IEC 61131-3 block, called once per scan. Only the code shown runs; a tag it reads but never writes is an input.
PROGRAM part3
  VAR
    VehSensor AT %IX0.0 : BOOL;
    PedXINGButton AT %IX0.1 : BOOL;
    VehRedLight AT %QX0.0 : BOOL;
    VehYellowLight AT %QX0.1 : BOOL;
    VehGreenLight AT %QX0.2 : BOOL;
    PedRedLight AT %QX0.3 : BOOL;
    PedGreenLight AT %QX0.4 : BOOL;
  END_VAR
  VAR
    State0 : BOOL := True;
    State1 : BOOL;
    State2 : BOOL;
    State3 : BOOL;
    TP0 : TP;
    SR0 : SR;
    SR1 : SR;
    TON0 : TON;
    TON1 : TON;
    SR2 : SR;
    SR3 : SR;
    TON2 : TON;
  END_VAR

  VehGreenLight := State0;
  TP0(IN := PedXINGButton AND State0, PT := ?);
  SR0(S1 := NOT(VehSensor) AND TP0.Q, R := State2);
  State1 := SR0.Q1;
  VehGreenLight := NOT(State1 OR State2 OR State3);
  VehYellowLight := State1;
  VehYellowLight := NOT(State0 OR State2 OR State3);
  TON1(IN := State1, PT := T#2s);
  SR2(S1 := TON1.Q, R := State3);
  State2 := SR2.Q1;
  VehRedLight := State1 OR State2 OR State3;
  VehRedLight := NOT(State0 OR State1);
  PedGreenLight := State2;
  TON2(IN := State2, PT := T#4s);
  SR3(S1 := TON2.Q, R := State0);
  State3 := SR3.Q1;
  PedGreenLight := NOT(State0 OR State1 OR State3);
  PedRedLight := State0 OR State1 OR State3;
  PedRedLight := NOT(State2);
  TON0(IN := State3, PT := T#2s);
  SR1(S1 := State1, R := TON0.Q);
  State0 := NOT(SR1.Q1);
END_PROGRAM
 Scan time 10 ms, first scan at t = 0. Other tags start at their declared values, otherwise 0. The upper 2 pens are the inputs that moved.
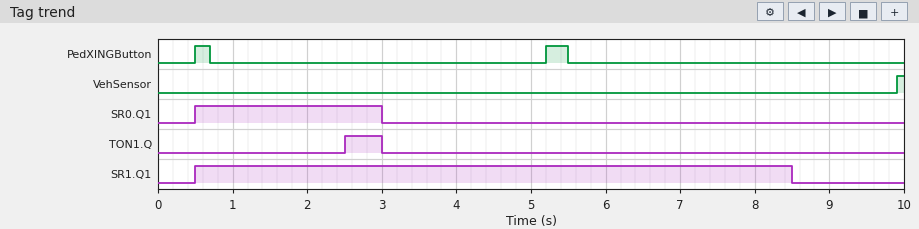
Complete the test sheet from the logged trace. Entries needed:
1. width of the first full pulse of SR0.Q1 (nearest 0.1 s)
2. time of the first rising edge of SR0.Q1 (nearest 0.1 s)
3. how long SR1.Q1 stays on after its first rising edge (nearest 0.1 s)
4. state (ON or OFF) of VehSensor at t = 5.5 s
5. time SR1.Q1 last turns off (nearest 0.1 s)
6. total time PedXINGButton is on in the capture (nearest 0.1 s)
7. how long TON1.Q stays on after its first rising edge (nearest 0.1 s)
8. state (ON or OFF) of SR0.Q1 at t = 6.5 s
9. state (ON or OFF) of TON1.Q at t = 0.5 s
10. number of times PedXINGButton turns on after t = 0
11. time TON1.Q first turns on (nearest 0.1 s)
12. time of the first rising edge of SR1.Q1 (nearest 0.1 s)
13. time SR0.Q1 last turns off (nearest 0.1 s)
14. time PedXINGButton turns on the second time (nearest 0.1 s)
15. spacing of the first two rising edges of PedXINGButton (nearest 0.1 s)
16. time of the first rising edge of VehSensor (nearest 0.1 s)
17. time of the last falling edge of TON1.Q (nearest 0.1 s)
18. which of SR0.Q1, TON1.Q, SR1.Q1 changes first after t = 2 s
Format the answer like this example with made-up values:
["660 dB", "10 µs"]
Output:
["2.5 s", "0.5 s", "8.0 s", "OFF", "8.5 s", "0.5 s", "0.5 s", "OFF", "OFF", "2", "2.5 s", "0.5 s", "3.0 s", "5.2 s", "4.7 s", "9.9 s", "3.0 s", "TON1.Q"]
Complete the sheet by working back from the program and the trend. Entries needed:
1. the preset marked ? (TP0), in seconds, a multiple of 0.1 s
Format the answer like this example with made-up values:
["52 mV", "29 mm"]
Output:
["2.5 s"]
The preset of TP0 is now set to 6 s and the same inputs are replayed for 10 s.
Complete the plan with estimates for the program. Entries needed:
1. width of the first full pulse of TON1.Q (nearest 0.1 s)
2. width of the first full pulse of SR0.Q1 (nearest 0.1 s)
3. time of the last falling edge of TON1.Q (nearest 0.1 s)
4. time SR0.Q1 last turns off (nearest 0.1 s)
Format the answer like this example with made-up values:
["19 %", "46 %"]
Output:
["4.0 s", "6.0 s", "6.5 s", "6.5 s"]
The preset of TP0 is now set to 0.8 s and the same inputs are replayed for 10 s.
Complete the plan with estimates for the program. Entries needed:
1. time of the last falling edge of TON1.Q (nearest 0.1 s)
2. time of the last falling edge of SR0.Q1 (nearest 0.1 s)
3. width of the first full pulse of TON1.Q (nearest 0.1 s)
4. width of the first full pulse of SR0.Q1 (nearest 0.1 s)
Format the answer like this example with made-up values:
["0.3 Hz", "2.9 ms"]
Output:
["2.5 s", "2.5 s", "0.0 s", "2.0 s"]
